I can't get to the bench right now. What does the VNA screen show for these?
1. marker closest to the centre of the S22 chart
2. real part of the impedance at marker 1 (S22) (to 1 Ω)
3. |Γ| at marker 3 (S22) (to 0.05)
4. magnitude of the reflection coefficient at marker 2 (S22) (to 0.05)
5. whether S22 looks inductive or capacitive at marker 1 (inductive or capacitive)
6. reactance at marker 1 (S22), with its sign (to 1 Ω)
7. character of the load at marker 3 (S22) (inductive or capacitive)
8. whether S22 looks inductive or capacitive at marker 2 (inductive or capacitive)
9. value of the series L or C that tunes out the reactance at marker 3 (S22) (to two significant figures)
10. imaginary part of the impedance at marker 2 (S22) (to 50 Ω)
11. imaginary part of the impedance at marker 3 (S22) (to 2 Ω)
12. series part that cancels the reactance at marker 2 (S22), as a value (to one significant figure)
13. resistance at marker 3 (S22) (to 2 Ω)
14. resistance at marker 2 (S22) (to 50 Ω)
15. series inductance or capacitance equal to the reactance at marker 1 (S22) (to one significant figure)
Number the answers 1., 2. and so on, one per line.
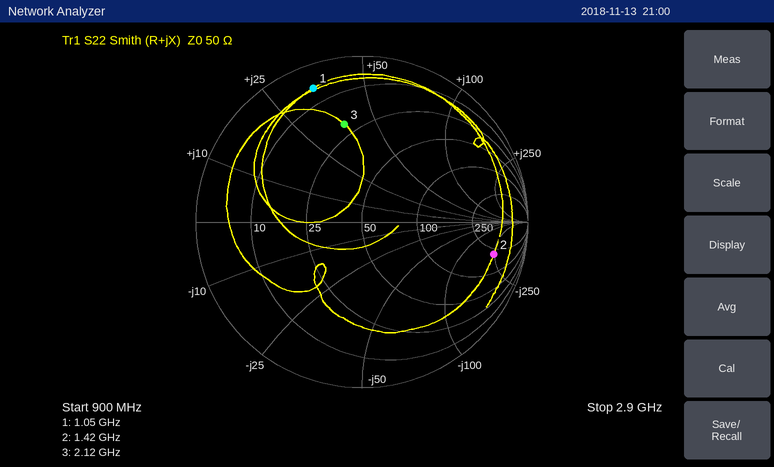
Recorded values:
1. marker 3
2. 6 Ω
3. 0.60
4. 0.80
5. inductive
6. +35 Ω
7. inductive
8. capacitive
9. 2.0 pF
10. -250 Ω
11. +38 Ω
12. 30 nH
13. 20 Ω
14. 200 Ω
15. 5 nH
